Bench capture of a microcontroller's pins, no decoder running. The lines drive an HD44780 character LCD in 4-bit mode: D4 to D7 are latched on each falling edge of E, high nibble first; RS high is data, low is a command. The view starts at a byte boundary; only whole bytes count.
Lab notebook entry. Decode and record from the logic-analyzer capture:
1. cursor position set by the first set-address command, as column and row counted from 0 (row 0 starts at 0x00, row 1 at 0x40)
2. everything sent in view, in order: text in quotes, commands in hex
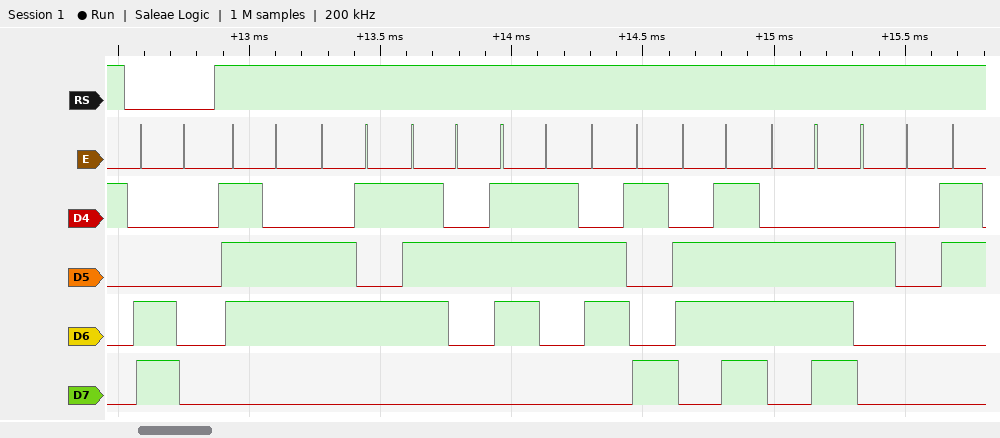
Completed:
column 0, row 1
0xC0 "version "
